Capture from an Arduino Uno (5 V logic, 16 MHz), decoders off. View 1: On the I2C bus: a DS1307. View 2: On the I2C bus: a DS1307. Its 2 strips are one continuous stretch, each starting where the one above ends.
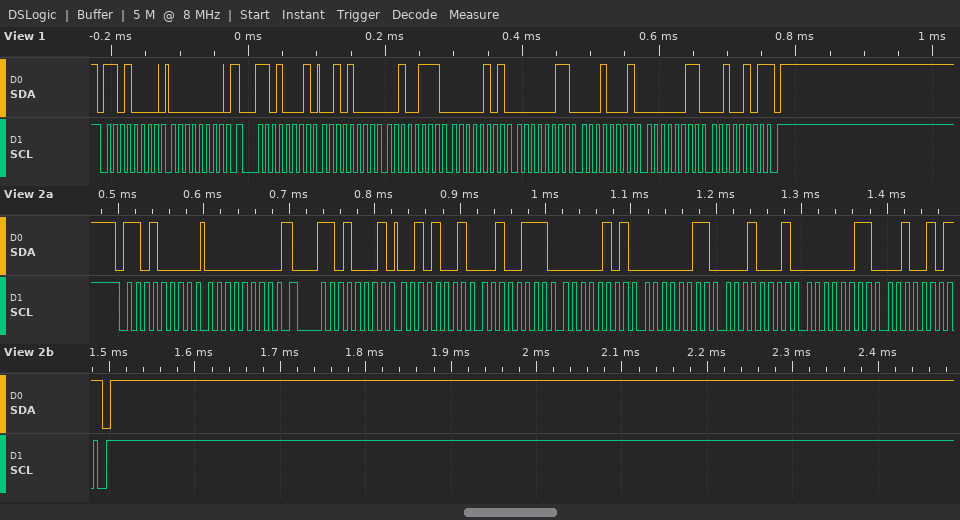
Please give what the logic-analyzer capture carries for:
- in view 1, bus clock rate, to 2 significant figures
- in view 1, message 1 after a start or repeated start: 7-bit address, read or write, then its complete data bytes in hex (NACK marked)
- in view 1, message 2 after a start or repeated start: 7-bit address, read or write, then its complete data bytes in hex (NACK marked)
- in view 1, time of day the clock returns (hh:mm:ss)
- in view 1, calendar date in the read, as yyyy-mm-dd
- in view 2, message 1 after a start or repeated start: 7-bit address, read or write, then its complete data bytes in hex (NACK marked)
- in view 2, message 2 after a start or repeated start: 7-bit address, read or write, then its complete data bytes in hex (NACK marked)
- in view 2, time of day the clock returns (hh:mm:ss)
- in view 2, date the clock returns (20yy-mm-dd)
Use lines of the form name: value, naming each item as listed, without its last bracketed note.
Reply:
in view 1, bus clock rate, to 2 significant figures: 100 kHz
in view 1, message 1 after a start or repeated start: 7-bit address, read or write, then its complete data bytes in hex: 0x68 write: 00
in view 1, message 2 after a start or repeated start: 7-bit address, read or write, then its complete data bytes in hex: 0x68 read: 28 27 05 03 11 03 25 NACK
in view 1, time of day the clock returns: 05:27:28
in view 1, calendar date in the read, as yyyy-mm-dd: 2025-03-11
in view 2, message 1 after a start or repeated start: 7-bit address, read or write, then its complete data bytes in hex: 0x68 write: 00
in view 2, message 2 after a start or repeated start: 7-bit address, read or write, then its complete data bytes in hex: 0x68 read: 29 27 05 03 11 03 25 NACK
in view 2, time of day the clock returns: 05:27:29
in view 2, date the clock returns: 2025-03-11
